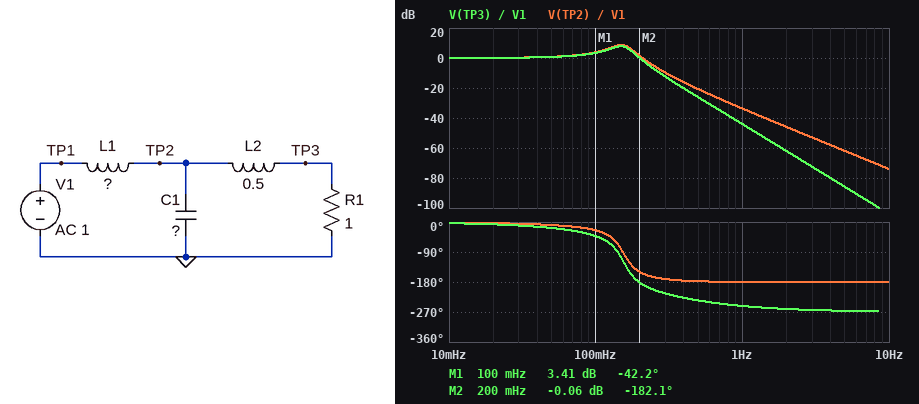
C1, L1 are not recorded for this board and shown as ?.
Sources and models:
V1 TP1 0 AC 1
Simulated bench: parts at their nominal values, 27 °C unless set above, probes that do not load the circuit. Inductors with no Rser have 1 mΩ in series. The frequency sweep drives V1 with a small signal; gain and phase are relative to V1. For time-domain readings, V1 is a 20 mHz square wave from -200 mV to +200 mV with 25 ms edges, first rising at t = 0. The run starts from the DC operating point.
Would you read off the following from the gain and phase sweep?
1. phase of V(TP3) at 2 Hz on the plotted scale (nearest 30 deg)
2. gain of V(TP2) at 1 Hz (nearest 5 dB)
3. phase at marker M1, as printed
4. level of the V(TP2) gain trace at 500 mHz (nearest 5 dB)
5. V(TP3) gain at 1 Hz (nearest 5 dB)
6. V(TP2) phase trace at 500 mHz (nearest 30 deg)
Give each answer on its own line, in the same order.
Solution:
-270 deg
-35 dB
-42.2 deg
-20 dB
-45 dB
-180 deg
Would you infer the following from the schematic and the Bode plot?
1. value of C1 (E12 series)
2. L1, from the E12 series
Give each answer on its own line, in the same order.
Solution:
2.7 F
470 mH
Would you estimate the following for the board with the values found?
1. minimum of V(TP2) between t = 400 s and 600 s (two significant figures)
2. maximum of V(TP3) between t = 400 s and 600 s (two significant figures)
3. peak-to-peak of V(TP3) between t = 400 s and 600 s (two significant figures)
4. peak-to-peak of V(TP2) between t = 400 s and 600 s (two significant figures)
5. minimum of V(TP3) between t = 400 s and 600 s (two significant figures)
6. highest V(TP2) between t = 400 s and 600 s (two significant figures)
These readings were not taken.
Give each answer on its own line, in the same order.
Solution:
-410 mV
390 mV
780 mV
830 mV
-390 mV
410 mV
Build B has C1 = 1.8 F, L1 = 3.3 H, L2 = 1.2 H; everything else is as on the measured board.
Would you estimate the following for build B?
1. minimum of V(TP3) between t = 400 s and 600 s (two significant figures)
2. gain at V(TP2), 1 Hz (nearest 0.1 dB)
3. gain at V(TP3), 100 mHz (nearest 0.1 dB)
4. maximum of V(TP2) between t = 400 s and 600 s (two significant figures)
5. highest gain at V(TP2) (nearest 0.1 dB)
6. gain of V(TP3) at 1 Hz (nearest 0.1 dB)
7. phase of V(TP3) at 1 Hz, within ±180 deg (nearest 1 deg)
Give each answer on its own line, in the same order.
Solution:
-200 mV
-47.3 dB
-4.7 dB
200 mV
0 dB
-64.9 dB
98 deg
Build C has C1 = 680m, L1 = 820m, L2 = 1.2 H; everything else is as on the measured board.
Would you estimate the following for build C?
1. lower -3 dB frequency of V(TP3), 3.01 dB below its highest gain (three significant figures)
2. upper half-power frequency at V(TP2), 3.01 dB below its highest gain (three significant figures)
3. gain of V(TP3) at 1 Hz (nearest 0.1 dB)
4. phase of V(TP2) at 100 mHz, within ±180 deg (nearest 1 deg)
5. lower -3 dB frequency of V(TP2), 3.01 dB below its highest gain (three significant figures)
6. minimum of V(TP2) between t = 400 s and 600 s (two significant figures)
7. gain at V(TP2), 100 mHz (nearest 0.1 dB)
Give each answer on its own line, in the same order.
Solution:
234 mHz
290 mHz
-43.8 dB
-18 deg
240 mHz
-350 mV
-0.7 dB
